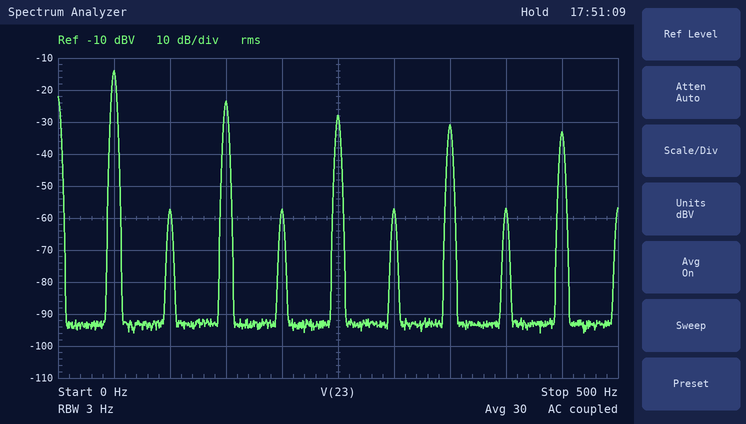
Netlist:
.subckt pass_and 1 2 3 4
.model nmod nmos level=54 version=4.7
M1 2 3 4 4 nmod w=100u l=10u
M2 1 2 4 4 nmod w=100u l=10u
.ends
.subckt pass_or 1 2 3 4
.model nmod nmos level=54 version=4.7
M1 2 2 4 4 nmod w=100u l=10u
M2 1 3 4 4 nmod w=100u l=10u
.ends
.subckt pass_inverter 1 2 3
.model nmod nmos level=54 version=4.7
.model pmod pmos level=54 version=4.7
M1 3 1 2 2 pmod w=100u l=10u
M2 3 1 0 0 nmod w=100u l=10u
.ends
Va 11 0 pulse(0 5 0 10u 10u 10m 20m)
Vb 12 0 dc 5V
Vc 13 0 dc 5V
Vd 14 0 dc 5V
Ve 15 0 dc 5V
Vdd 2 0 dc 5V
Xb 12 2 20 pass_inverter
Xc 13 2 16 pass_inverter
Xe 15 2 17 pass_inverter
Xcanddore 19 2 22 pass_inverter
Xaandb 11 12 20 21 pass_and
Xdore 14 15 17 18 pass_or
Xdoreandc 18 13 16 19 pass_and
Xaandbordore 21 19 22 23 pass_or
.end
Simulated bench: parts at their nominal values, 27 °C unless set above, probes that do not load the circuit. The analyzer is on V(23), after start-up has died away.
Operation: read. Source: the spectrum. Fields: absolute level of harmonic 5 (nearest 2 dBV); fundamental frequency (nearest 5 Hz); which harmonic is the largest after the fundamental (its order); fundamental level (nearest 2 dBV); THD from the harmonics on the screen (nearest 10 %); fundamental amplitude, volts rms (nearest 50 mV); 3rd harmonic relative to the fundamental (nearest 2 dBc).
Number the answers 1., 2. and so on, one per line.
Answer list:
1. -28 dBV
2. 50 Hz
3. 3
4. -14 dBV
5. 40 %
6. 200 mV
7. -10 dBc
